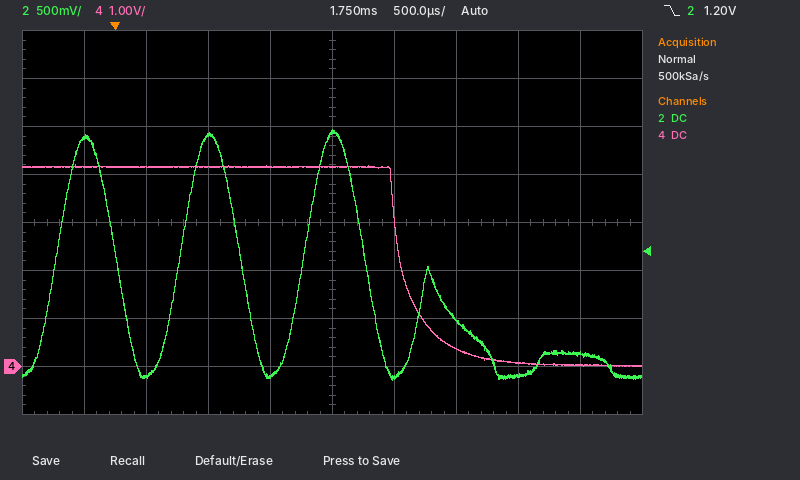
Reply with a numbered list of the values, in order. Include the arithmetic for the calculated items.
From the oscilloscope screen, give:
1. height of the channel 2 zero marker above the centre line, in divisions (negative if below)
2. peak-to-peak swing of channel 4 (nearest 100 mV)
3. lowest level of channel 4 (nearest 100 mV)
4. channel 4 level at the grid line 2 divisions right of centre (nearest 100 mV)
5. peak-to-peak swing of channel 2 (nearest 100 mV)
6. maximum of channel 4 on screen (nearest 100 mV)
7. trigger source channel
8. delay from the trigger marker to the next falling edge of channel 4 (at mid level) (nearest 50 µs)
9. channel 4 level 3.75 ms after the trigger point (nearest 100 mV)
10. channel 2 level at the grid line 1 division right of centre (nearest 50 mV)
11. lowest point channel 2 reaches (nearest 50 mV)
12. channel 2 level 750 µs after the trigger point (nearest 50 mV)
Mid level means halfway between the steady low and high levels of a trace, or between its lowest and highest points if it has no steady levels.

1. -3.0 div
2. 4.2 V − (0.0 V) = 4.2 V
3. 0.0 V
4. 400 mV
5. 2.60 V
6. 4.2 V
7. channel 2
8. 2.30 ms
9. 0.0 V
10. -100 mV
11. -150 mV
12. 2.40 V
